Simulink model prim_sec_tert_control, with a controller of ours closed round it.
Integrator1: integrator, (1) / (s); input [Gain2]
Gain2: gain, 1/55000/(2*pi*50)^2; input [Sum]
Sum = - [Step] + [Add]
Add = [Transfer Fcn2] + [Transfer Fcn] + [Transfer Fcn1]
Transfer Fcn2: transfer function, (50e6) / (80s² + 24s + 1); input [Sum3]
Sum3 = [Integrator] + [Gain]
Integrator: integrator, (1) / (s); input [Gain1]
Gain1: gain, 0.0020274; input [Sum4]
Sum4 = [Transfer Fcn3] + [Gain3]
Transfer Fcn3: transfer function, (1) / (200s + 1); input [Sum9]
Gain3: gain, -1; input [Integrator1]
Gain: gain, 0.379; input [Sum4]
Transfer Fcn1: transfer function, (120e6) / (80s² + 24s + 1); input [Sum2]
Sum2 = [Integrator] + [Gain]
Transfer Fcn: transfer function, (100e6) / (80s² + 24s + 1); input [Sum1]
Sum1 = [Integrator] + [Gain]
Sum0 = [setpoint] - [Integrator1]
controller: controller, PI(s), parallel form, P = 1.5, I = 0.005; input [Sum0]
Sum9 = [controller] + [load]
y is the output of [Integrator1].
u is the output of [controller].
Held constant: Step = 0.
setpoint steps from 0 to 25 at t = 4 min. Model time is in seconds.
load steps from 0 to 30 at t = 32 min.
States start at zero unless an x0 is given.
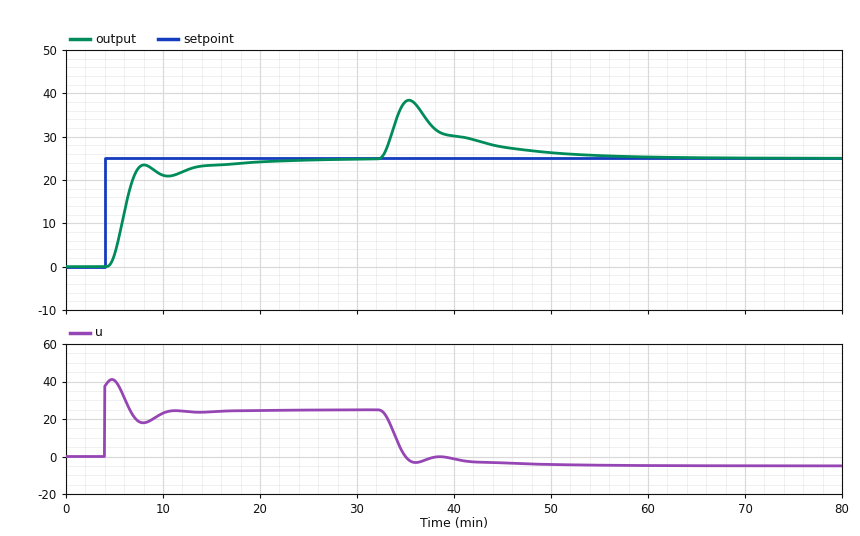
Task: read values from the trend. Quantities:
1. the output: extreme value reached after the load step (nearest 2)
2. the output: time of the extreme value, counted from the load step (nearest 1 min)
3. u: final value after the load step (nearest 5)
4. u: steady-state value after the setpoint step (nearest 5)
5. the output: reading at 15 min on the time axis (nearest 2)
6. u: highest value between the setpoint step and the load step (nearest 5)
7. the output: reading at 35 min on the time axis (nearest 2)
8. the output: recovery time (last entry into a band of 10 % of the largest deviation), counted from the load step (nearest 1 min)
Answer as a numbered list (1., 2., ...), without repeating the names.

1. 38
2. 3 min
3. -5
4. 25
5. 24
6. 40
7. 38
8. 18 min
